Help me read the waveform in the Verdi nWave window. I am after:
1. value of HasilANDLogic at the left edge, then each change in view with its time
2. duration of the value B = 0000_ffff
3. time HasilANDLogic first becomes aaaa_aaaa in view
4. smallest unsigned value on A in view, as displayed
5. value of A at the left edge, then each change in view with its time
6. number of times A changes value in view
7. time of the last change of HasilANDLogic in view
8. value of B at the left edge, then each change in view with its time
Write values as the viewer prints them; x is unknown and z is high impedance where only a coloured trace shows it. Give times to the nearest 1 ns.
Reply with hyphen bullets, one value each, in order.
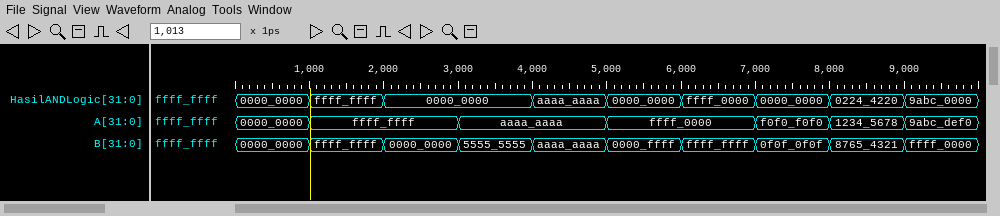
- 0000_0000, ffff_ffff at 1 ns, 0000_0000 at 2 ns, aaaa_aaaa at 4 ns, 0000_0000 at 5 ns, ffff_0000 at 6 ns, 0000_0000 at 7 ns, 0224_4220 at 8 ns, 9abc_0000 at 9 ns
- 1 ns
- 4 ns
- 0000_0000
- 0000_0000, ffff_ffff at 1 ns, aaaa_aaaa at 3 ns, ffff_0000 at 5 ns, f0f0_f0f0 at 7 ns, 1234_5678 at 8 ns, 9abc_def0 at 9 ns
- 6
- 9 ns
- 0000_0000, ffff_ffff at 1 ns, 0000_0000 at 2 ns, 5555_5555 at 3 ns, aaaa_aaaa at 4 ns, 0000_ffff at 5 ns, ffff_ffff at 6 ns, 0f0f_0f0f at 7 ns, 8765_4321 at 8 ns, ffff_0000 at 9 ns
